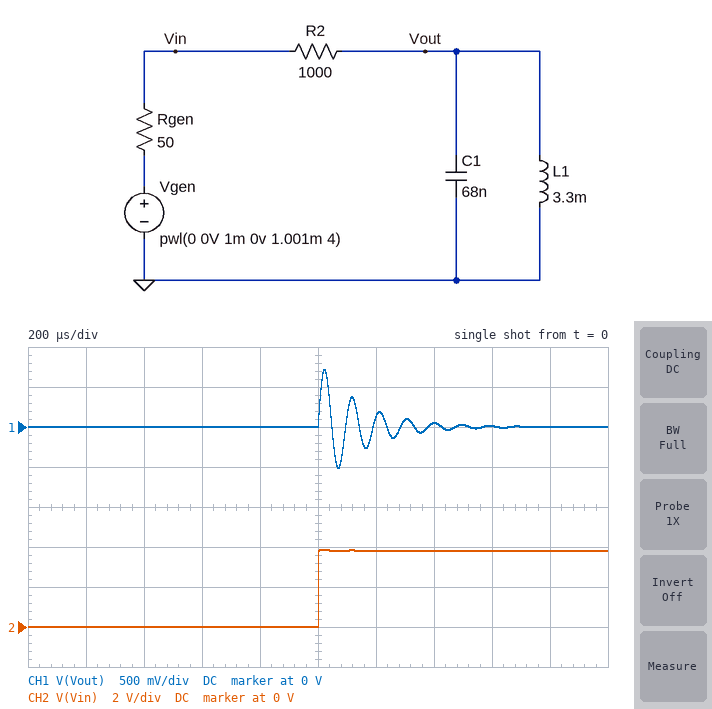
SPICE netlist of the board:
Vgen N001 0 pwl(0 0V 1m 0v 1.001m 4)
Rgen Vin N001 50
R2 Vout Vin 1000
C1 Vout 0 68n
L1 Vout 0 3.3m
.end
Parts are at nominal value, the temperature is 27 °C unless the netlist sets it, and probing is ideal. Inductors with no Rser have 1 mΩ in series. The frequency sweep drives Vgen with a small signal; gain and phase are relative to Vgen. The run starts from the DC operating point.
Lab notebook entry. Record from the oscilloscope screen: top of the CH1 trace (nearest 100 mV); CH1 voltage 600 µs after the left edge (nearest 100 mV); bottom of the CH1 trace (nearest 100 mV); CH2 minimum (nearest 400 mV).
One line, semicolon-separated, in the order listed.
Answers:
700 mV; 0 V; -500 mV; 0 V
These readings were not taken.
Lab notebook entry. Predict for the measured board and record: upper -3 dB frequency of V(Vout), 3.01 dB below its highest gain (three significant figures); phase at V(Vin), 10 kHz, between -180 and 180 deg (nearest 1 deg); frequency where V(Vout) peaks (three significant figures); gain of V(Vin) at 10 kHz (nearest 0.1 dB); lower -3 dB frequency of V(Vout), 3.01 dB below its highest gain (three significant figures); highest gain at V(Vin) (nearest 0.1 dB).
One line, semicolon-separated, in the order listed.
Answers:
11.8 kHz; 1 deg; 10.6 kHz; -0.1 dB; 9.57 kHz; 0 dB
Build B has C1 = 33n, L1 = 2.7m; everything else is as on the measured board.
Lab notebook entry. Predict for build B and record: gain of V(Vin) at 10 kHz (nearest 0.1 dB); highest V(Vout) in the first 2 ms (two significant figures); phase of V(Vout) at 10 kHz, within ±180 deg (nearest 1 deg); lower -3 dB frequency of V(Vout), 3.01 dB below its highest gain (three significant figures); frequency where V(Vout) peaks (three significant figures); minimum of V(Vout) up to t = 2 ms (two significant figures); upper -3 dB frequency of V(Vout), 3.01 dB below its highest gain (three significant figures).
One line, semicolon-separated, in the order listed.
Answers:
-0.4 dB; 890 mV; 76 deg; 14.7 kHz; 16.9 kHz; -580 mV; 19.3 kHz
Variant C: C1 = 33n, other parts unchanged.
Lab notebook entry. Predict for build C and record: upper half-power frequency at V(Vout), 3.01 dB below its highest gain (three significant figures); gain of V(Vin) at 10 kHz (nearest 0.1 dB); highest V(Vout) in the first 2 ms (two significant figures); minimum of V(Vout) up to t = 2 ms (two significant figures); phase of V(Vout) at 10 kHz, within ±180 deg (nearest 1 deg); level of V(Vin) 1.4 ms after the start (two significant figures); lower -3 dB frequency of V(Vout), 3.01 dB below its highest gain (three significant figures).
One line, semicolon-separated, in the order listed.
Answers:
17.7 kHz; -0.4 dB; 970 mV; -600 mV; 71 deg; 3.8 V; 13.1 kHz
